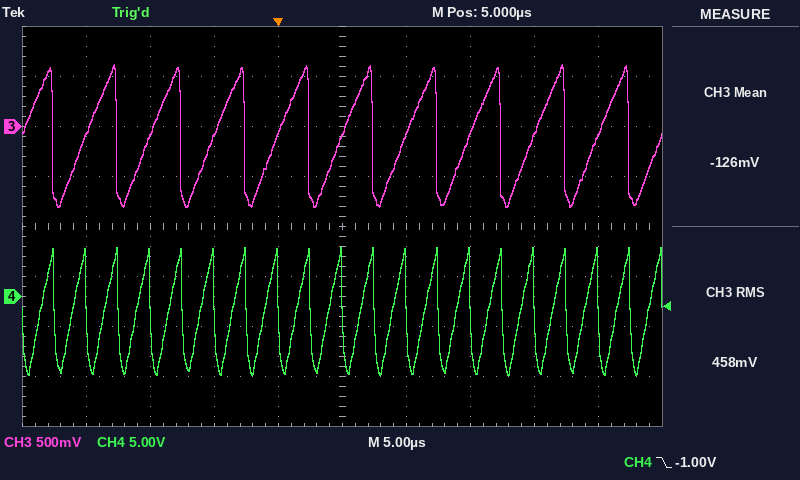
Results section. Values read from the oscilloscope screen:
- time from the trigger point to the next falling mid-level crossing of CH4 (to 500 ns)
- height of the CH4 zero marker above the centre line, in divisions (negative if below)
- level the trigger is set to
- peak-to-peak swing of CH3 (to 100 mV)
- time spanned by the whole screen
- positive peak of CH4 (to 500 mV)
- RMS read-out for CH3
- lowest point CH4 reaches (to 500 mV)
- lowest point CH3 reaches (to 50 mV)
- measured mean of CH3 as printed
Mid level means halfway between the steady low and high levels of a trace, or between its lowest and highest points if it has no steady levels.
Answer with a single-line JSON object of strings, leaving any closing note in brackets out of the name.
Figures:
{"time from the trigger point to the next falling mid-level crossing of CH4": "2.5 µs", "height of the CH4 zero marker above the centre line, in divisions": "-1.4 div", "level the trigger is set to": "-1.00 V", "peak-to-peak swing of CH3": "1.40 V", "time spanned by the whole screen": "50 µs", "positive peak of CH4": "5.0 V", "RMS read-out for CH3": "458 mV", "lowest point CH4 reaches": "-8.0 V", "lowest point CH3 reaches": "-800 mV", "measured mean of CH3 as printed": "-126 mV"}
